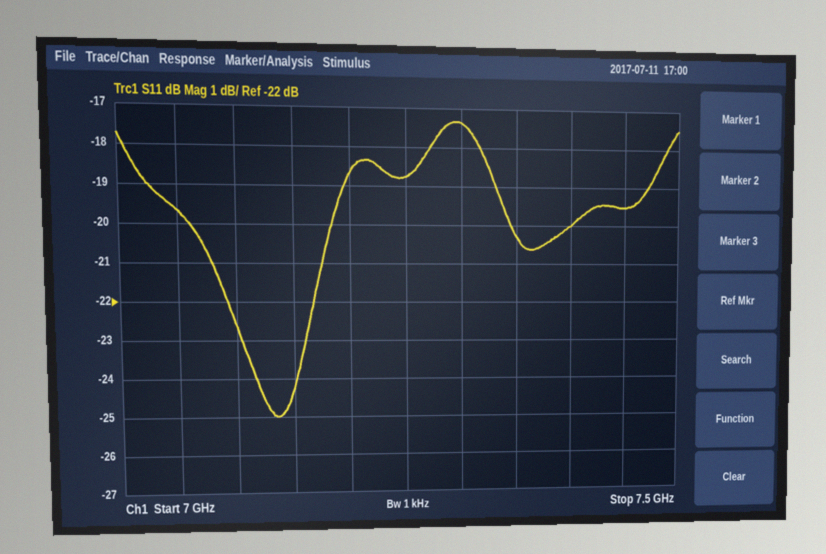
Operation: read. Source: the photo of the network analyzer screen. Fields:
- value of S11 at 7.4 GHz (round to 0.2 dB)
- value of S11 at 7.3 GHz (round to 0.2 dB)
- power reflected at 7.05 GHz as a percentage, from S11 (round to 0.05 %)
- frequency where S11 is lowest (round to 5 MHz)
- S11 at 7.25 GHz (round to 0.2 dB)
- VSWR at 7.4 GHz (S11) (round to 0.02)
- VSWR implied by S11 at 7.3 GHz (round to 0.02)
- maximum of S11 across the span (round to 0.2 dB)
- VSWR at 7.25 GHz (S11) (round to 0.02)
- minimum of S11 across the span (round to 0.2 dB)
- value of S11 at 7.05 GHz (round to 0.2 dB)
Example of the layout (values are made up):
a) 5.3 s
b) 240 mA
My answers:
a) -20.0 dB
b) -17.4 dB
c) 1.10 %
d) 7.135 GHz
e) -18.8 dB
f) 1.22
g) 1.32
h) -17.4 dB
i) 1.26
j) -25.0 dB
k) -19.6 dB
